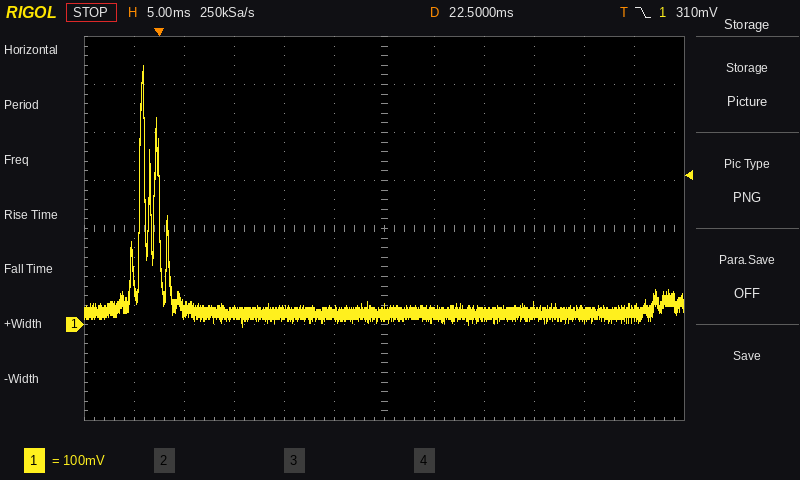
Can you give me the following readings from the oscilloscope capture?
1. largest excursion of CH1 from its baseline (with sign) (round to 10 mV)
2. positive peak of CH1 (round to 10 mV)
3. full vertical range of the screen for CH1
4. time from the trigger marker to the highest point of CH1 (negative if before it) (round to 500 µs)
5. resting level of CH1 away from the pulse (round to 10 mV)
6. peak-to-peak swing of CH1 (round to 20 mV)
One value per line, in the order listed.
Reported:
+520 mV
540 mV
800 mV
-1.5 ms
20 mV
540 mV
